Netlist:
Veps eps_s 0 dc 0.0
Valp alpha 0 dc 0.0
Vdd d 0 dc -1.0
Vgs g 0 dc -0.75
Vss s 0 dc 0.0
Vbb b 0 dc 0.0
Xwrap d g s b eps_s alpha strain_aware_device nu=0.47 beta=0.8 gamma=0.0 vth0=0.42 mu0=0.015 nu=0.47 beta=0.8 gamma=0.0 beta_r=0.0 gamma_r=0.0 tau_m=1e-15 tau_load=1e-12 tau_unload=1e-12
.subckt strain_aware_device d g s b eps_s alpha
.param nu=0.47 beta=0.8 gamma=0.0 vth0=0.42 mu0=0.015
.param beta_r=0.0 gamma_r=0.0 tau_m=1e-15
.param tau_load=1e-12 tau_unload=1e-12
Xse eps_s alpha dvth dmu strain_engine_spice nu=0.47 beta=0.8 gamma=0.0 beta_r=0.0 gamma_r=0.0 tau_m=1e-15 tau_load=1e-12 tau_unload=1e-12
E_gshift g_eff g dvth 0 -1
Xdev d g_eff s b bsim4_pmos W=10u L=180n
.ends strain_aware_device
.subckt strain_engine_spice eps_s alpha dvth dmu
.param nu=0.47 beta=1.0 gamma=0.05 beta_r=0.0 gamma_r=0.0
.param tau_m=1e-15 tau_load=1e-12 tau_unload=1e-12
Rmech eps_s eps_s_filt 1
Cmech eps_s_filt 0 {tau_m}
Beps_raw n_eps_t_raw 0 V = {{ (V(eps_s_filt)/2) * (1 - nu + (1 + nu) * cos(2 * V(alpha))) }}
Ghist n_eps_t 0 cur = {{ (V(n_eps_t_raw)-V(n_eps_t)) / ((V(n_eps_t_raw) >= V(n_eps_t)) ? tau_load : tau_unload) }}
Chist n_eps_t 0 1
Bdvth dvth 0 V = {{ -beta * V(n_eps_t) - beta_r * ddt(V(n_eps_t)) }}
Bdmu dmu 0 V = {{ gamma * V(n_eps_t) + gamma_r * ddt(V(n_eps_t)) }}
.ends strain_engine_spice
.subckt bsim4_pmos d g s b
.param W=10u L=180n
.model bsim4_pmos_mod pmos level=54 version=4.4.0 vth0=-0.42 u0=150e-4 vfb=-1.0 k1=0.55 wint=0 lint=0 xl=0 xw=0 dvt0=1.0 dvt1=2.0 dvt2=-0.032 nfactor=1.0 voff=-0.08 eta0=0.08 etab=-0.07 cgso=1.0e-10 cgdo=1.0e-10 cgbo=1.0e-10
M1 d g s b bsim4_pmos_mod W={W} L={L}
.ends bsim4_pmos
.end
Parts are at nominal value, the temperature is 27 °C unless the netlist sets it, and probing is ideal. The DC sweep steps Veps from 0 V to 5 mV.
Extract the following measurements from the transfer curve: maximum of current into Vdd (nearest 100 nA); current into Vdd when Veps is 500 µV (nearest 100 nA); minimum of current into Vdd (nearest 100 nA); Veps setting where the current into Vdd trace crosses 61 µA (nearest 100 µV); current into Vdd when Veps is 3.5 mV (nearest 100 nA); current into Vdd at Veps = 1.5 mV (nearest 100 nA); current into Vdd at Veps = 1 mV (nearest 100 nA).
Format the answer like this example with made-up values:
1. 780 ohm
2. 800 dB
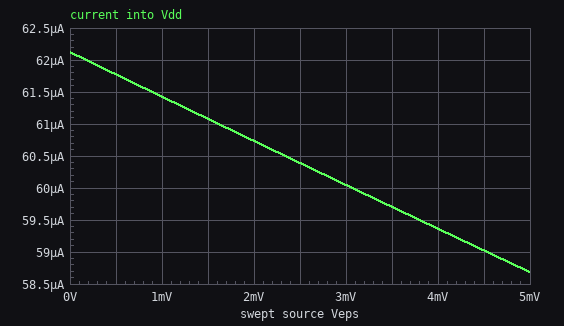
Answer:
1. 62.1 µA
2. 61.8 µA
3. 58.7 µA
4. 1.6 mV
5. 59.7 µA
6. 61.1 µA
7. 61.4 µA
